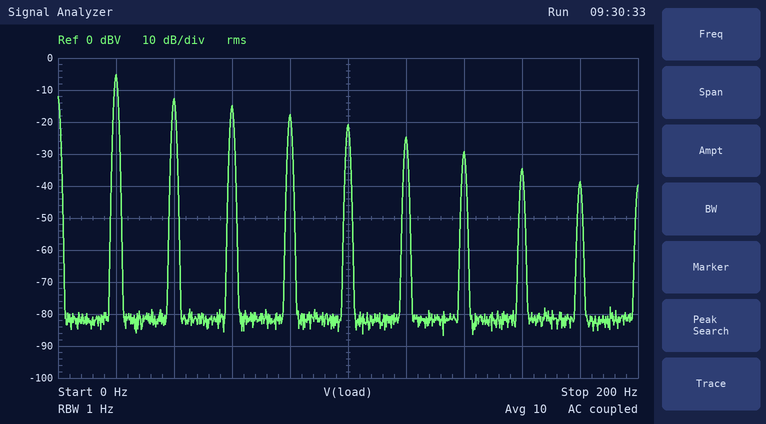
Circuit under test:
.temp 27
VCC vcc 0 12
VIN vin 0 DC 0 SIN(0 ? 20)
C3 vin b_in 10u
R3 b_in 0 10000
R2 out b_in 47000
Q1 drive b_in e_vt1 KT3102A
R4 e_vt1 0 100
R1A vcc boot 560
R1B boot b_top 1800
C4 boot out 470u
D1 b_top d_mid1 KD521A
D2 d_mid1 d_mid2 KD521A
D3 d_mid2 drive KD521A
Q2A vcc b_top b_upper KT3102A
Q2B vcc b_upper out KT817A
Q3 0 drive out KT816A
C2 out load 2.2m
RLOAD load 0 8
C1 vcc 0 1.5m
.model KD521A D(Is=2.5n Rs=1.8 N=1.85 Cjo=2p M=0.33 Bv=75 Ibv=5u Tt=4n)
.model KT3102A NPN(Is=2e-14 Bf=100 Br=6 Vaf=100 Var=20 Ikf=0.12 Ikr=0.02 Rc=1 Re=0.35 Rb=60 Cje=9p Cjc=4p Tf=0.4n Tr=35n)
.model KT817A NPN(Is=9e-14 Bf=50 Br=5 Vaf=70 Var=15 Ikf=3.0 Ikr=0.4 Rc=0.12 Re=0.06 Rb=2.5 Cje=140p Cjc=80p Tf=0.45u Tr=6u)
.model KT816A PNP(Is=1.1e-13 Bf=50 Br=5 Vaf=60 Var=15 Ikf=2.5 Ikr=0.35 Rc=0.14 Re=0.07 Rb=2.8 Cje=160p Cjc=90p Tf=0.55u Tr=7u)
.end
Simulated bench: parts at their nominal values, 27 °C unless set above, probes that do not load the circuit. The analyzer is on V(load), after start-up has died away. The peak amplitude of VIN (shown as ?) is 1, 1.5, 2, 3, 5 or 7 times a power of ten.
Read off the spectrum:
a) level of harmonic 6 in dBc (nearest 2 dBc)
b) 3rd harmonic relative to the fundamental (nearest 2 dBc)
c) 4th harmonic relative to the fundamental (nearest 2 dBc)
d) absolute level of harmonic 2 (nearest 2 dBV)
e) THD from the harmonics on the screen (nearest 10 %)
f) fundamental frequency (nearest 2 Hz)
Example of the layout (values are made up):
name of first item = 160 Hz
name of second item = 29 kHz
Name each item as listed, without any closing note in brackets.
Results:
level of harmonic 6 in dBc = -20 dBc
3rd harmonic relative to the fundamental = -10 dBc
4th harmonic relative to the fundamental = -12 dBc
absolute level of harmonic 2 = -12 dBV
THD from the harmonics on the screen = 60 %
fundamental frequency = 20 Hz
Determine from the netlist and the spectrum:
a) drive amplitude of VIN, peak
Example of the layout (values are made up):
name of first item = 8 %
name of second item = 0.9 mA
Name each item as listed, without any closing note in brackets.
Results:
drive amplitude of VIN, peak = 100 mV
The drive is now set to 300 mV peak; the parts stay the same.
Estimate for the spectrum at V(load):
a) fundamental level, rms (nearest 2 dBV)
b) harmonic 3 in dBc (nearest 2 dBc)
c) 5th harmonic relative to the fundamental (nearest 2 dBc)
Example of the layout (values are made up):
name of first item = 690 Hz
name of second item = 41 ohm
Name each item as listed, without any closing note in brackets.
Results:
fundamental level, rms = 4 dBV
harmonic 3 in dBc = -12 dBc
5th harmonic relative to the fundamental = -24 dBc
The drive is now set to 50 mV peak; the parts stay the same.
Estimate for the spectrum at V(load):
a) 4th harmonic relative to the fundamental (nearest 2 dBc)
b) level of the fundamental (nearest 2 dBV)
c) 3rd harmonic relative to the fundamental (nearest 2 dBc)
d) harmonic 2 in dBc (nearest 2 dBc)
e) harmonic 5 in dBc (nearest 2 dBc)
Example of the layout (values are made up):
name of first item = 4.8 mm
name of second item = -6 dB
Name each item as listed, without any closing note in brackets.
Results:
4th harmonic relative to the fundamental = -26 dBc
level of the fundamental = -14 dBV
3rd harmonic relative to the fundamental = -20 dBc
harmonic 2 in dBc = -14 dBc
harmonic 5 in dBc = -32 dBc
